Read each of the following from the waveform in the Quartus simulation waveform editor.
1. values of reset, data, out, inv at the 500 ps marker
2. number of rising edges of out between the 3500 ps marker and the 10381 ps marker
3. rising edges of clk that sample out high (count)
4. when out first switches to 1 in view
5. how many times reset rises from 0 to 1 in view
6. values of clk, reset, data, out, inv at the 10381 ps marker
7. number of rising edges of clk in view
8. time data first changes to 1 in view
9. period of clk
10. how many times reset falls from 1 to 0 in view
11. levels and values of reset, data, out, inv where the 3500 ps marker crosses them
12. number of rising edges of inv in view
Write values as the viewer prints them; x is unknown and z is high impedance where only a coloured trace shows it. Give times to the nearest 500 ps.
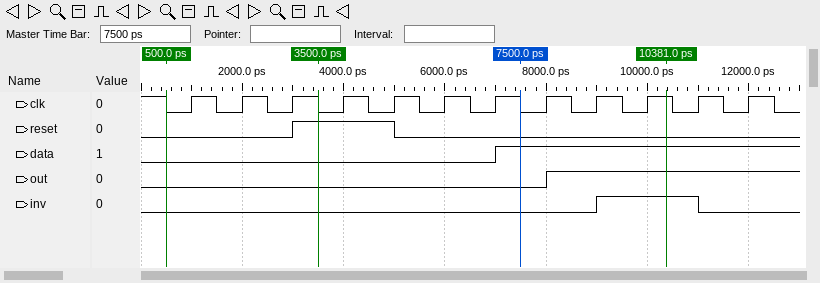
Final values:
reset=0, data=0, out=0, inv=0
1
4
8000 ps
1
clk=1, reset=0, data=1, out=1, inv=1
12
7000 ps
1000 ps
1
reset=1, data=0, out=0, inv=0
1
